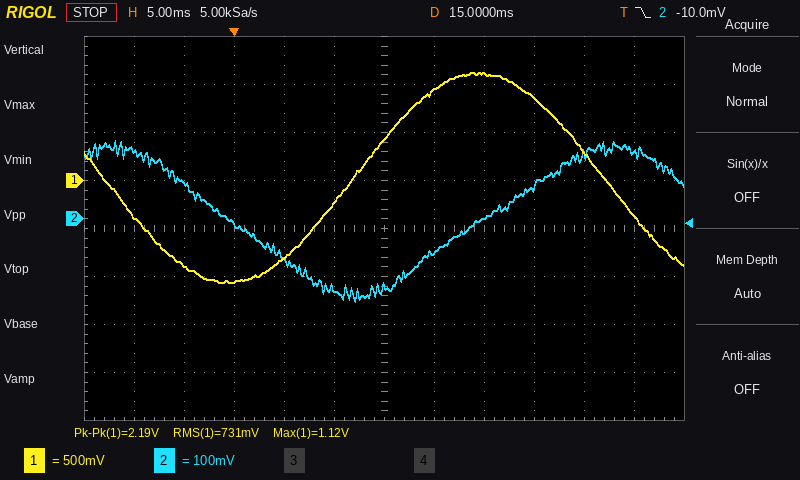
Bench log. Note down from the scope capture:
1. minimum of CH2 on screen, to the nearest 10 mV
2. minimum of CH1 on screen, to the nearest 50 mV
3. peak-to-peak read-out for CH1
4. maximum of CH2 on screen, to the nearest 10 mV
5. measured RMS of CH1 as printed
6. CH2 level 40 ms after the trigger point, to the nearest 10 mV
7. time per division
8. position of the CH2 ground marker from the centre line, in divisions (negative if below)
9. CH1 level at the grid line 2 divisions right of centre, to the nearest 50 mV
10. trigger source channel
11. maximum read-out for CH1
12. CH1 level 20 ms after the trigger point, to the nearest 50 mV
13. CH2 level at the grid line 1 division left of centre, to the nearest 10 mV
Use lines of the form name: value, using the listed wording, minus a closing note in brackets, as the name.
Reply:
minimum of CH2 on screen, to the nearest 10 mV: -170 mV
minimum of CH1 on screen, to the nearest 50 mV: -1.05 V
peak-to-peak read-out for CH1: 2.19 V
maximum of CH2 on screen, to the nearest 10 mV: 160 mV
measured RMS of CH1 as printed: 731 mV
CH2 level 40 ms after the trigger point, to the nearest 10 mV: 140 mV
time per division: 5 ms
position of the CH2 ground marker from the centre line, in divisions: +0.2 div
CH1 level at the grid line 2 divisions right of centre, to the nearest 50 mV: 1.10 V
trigger source channel: CH2
maximum read-out for CH1: 1.12 V
CH1 level 20 ms after the trigger point, to the nearest 50 mV: 950 mV
CH2 level at the grid line 1 division left of centre, to the nearest 10 mV: -140 mV
